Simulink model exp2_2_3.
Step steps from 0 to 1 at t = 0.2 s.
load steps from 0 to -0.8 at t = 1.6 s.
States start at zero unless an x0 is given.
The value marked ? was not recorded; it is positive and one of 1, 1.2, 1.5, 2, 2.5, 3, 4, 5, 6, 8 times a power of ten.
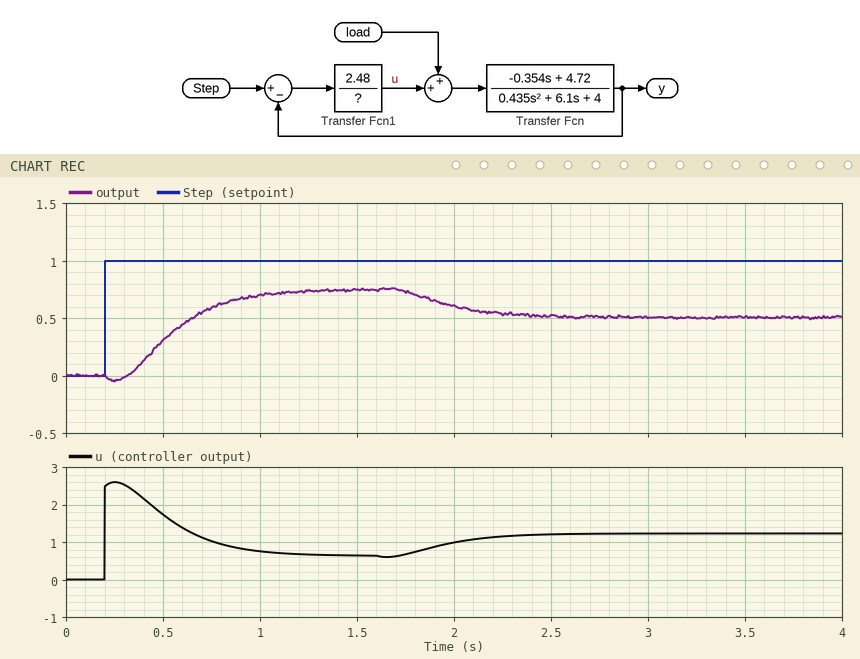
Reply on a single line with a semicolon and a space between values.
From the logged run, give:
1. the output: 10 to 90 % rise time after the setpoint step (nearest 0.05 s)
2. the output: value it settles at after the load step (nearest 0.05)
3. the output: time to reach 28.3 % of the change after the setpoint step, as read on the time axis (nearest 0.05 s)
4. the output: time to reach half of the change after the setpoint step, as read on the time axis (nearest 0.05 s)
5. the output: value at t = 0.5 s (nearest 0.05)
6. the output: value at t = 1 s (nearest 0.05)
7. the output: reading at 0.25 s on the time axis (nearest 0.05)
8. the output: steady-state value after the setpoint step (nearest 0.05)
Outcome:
0.55 s; 0.50; 0.45 s; 0.55 s; 0.30; 0.70; -0.05; 0.75
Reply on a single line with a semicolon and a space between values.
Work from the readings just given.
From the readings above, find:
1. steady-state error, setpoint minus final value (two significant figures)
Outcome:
0.25
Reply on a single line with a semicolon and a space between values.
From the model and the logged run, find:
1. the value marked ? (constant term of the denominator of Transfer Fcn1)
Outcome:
1
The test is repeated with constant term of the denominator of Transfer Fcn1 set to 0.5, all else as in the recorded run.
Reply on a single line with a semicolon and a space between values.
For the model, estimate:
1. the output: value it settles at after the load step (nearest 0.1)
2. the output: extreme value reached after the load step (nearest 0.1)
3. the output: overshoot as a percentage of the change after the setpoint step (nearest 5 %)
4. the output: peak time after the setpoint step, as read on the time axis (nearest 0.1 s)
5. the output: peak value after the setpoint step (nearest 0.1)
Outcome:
0.7; 0.7; 10 %; 0.8 s; 0.9
